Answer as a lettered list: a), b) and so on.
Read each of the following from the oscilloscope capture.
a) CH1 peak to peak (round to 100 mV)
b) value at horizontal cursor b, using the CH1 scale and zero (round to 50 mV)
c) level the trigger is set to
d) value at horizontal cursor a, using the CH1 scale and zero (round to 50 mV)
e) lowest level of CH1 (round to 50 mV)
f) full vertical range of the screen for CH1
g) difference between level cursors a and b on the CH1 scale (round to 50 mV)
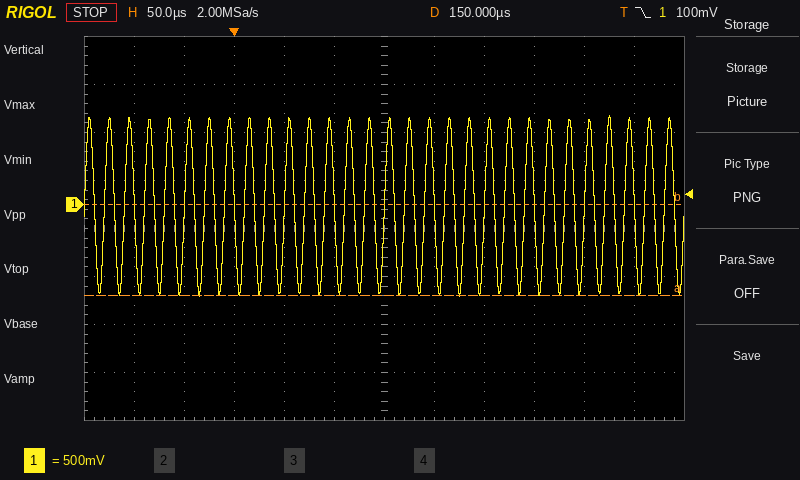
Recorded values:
a) 1.90 V
b) 0 mV
c) 100 mV
d) -950 mV
e) -950 mV
f) 4 V
g) 950 mV
